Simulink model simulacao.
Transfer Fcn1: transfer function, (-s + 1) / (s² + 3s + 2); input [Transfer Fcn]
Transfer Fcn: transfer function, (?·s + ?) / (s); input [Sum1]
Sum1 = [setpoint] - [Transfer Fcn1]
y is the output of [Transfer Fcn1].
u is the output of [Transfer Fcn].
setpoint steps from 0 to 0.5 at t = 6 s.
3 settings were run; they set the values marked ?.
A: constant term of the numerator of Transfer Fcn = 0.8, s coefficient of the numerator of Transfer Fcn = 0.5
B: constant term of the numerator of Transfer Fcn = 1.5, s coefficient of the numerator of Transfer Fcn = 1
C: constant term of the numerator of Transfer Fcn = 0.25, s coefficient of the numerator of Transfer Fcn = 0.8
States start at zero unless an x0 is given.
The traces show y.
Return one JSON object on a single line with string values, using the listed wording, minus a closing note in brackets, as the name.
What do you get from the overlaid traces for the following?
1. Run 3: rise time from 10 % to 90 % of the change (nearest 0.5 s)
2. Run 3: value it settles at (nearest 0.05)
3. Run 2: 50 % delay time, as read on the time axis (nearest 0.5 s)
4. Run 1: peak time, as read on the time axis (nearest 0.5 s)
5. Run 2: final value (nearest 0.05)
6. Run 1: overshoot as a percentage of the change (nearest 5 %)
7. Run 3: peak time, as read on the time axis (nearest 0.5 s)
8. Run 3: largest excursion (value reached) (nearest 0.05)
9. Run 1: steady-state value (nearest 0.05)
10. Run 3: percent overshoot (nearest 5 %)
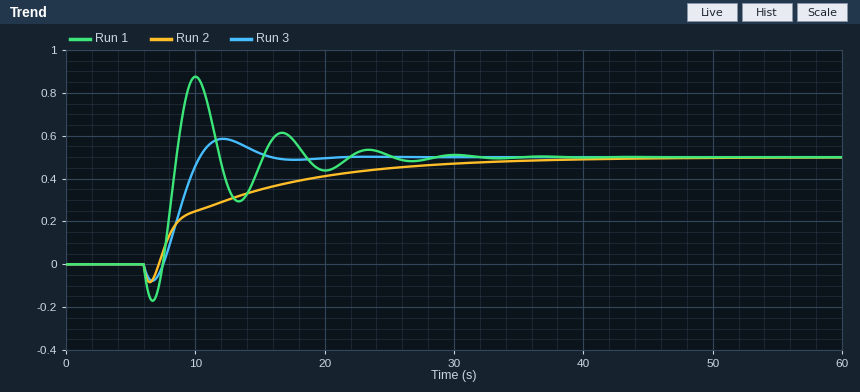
{"Run 3: rise time from 10 % to 90 % of the change": "2.0 s", "Run 3: value it settles at": "0.50", "Run 2: 50 % delay time, as read on the time axis": "10.0 s", "Run 1: peak time, as read on the time axis": "10.0 s", "Run 2: final value": "0.50", "Run 1: overshoot as a percentage of the change": "75 %", "Run 3: peak time, as read on the time axis": "12.0 s", "Run 3: largest excursion (value reached)": "0.60", "Run 1: steady-state value": "0.50", "Run 3: percent overshoot": "15 %"}
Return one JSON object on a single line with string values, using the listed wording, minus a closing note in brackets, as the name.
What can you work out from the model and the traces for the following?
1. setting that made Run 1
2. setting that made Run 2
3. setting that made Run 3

{"setting that made Run 1": "B", "setting that made Run 2": "C", "setting that made Run 3": "A"}
